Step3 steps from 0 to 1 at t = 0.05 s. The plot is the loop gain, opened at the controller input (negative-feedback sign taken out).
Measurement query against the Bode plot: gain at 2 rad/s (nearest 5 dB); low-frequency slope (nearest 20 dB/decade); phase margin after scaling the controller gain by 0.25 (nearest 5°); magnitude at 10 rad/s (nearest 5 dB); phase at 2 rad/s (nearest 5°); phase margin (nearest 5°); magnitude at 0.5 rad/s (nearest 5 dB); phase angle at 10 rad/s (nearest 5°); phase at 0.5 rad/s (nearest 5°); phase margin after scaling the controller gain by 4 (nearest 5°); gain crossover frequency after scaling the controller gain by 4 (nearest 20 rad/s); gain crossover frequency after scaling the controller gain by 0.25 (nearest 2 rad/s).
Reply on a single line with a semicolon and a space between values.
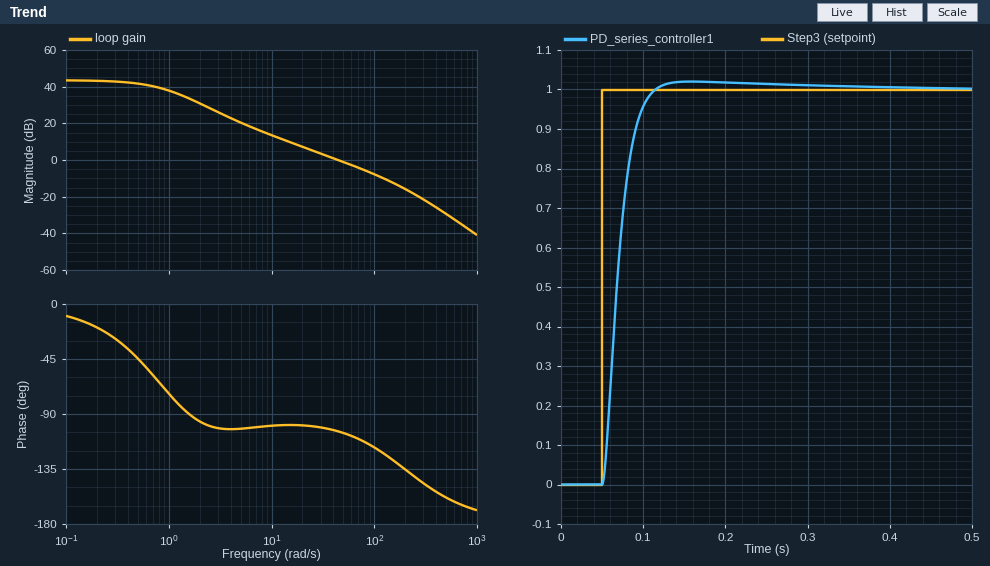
30 dB; 0 dB/decade; 80°; 15 dB; -95°; 75°; 40 dB; -100°; -45°; 55°; 140 rad/s; 12 rad/s
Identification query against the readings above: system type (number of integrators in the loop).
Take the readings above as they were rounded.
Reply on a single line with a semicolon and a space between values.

0
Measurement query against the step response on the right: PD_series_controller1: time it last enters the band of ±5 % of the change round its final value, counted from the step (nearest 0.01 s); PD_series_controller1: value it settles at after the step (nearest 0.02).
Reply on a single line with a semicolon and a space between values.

0.05 s; 1.00
